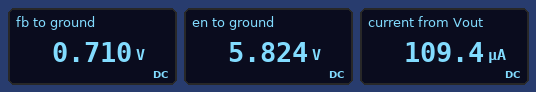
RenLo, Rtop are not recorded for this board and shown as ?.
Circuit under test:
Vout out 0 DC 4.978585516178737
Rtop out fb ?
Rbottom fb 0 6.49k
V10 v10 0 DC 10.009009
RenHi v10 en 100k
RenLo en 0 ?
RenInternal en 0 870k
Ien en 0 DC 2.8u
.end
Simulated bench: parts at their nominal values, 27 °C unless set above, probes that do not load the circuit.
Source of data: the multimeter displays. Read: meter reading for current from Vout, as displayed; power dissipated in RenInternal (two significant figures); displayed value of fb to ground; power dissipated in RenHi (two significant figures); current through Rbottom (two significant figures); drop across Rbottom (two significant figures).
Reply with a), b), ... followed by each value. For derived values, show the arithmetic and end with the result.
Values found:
a) 109.4 µA
b) (5.824 V)^2 / 870 kΩ = 39 µW
c) 0.710 V
d) (10.01 V - 5.824 V)^2 / 100 kΩ = 180 µW
e) (710 mV) / 6.49 kΩ = 110 µA
f) 710 mV = 710 mV
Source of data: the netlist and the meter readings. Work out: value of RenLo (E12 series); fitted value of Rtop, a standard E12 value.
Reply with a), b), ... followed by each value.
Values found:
a) 180 kΩ
b) 39 kΩ
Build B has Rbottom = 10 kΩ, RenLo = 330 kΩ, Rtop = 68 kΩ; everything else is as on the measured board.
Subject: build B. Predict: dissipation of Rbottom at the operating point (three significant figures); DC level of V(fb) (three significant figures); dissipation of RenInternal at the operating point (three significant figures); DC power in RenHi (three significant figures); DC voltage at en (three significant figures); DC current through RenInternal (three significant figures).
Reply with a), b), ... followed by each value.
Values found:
a) 40.7 µW
b) 638 mV
c) 54.1 µW
d) 99.1 µW
e) 6.86 V
f) 7.89 µA
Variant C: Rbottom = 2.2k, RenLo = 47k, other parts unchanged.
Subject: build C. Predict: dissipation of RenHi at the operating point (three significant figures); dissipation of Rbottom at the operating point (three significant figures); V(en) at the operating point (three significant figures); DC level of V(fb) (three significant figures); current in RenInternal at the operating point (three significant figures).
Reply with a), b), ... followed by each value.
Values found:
a) 491 µW
b) 32.1 µW
c) 3.00 V
d) 266 mV
e) 3.45 µA
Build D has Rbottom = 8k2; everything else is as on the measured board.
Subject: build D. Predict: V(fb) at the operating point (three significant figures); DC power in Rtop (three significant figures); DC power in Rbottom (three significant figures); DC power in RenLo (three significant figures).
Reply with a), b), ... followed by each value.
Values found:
a) 865 mV
b) 434 µW
c) 91.2 µW
d) 188 µW
